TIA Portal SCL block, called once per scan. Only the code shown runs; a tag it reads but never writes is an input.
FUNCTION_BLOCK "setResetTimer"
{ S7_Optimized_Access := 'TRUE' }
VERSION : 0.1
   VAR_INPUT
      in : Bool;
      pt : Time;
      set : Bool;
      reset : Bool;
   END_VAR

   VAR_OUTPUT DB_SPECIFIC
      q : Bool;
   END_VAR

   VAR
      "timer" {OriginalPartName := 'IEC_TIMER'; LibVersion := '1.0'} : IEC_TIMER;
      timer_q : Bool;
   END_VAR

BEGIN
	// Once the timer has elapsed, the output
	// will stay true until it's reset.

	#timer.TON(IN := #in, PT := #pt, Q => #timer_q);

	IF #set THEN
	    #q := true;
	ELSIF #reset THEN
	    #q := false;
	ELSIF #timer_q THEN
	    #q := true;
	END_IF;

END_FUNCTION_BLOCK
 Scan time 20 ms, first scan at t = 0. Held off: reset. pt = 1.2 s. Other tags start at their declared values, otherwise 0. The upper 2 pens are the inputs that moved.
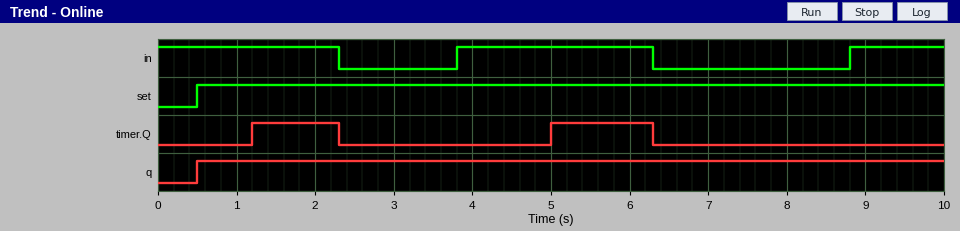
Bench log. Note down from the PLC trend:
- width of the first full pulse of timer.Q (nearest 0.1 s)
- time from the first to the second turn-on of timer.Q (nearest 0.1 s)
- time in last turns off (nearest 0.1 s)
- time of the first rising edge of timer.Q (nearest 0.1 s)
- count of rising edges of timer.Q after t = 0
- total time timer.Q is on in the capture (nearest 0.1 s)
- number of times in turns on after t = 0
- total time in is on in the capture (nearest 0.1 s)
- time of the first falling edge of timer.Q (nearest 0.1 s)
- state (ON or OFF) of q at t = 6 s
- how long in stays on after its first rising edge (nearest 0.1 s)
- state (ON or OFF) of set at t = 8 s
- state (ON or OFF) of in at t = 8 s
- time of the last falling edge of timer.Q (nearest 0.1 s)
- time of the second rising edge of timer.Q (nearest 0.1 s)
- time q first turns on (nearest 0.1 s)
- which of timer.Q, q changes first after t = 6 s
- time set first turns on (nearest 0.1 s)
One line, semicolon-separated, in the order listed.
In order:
1.1 s; 3.8 s; 6.3 s; 1.2 s; 2; 2.4 s; 2; 6.0 s; 2.3 s; ON; 2.5 s; ON; OFF; 6.3 s; 5.0 s; 0.5 s; timer.Q; 0.5 s
